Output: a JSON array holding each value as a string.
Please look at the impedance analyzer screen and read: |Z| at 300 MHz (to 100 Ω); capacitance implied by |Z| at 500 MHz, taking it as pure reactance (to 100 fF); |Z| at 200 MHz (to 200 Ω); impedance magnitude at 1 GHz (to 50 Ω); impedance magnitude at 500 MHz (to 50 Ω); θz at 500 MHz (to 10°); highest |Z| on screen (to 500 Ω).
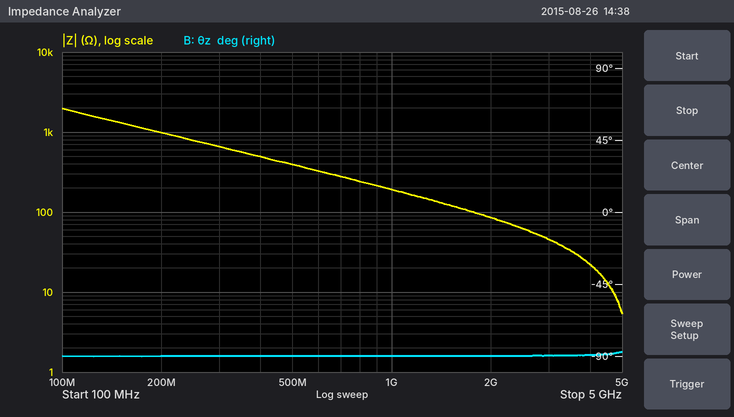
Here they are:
["700 Ω", "800 fF", "1.0 kΩ", "200 Ω", "400 Ω", "-90°", "2.0 kΩ"]
